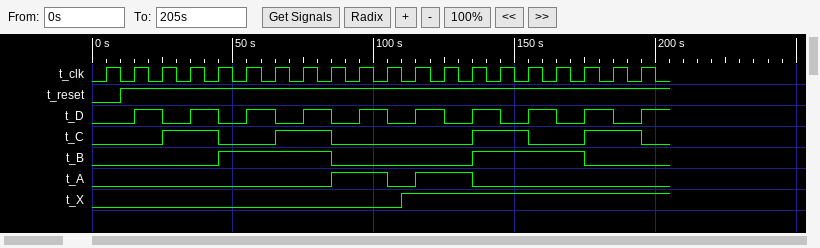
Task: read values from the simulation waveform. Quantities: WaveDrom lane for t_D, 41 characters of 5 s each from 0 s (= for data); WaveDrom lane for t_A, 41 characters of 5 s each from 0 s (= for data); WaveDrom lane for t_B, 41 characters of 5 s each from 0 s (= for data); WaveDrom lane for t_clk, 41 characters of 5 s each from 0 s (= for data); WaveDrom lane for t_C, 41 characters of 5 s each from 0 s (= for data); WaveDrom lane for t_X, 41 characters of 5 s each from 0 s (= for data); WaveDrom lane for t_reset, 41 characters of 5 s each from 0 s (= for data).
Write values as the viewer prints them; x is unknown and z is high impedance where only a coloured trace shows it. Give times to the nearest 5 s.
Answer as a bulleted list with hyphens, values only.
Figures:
- {name: 't_D', wave: '0..1.0.1.0.1.0.1.0.1.0.1.0.1.0.1.0.1.0.1.'}
- {name: 't_A', wave: '0................1...0.1...0.............'}
- {name: 't_B', wave: '0........1.......0.........1.......0.....'}
- {name: 't_clk', wave: '01010101010101010101010101010101010101010'}
- {name: 't_C', wave: '0....1...0...1...0.........1...0...1...0.'}
- {name: 't_X', wave: '0.....................1..................'}
- {name: 't_reset', wave: '0.1......................................'}
